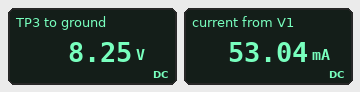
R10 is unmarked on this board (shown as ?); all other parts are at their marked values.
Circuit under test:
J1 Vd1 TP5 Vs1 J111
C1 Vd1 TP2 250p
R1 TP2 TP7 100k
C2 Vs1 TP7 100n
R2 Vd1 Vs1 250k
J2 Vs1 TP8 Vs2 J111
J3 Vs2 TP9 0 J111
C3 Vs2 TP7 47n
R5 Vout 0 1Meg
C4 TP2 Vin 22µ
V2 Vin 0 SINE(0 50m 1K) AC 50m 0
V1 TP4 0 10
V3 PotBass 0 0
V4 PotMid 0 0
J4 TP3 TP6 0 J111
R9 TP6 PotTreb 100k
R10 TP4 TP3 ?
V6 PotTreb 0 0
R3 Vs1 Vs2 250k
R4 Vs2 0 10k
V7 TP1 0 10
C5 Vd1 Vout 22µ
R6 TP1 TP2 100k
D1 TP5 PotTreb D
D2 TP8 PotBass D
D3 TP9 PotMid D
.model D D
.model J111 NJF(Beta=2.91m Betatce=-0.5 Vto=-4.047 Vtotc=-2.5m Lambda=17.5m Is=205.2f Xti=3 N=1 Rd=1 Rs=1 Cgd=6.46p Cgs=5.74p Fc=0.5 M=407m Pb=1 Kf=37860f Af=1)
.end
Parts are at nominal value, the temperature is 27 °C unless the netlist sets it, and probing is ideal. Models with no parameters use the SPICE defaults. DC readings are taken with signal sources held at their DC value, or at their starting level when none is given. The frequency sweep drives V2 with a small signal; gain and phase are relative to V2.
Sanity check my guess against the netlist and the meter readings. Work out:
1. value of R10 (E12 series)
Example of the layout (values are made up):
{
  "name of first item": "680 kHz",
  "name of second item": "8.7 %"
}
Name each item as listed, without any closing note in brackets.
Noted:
{
  "value of R10": "33 Ω"
}
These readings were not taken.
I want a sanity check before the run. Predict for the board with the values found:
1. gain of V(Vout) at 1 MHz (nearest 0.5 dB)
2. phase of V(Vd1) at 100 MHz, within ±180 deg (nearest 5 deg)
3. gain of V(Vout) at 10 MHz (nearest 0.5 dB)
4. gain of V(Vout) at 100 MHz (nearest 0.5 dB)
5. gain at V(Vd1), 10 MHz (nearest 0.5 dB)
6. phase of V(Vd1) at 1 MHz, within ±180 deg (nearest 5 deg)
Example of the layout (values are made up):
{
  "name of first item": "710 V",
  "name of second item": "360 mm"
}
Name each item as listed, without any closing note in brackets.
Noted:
{
  "gain of V(Vout) at 1 MHz": "-17.0 dB",
  "phase of V(Vd1) at 100 MHz, within ±180 deg": "5 deg",
  "gain of V(Vout) at 10 MHz": "-2.0 dB",
  "gain of V(Vout) at 100 MHz": "0 dB",
  "gain at V(Vd1), 10 MHz": "-2.0 dB",
  "phase of V(Vd1) at 1 MHz, within ±180 deg": "80 deg"
}
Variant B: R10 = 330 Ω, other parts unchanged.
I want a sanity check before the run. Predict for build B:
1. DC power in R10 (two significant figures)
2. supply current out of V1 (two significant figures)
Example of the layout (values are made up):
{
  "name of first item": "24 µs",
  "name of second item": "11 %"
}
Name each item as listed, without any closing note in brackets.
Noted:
{
  "DC power in R10": "230 mW",
  "supply current out of V1": "26 mA"
}
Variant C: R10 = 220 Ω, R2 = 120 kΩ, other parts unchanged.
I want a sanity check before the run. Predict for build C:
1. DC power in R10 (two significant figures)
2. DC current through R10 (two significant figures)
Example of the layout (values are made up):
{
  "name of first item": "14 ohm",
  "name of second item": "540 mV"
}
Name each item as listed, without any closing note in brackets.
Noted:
{
  "DC power in R10": "290 mW",
  "DC current through R10": "36 mA"
}
